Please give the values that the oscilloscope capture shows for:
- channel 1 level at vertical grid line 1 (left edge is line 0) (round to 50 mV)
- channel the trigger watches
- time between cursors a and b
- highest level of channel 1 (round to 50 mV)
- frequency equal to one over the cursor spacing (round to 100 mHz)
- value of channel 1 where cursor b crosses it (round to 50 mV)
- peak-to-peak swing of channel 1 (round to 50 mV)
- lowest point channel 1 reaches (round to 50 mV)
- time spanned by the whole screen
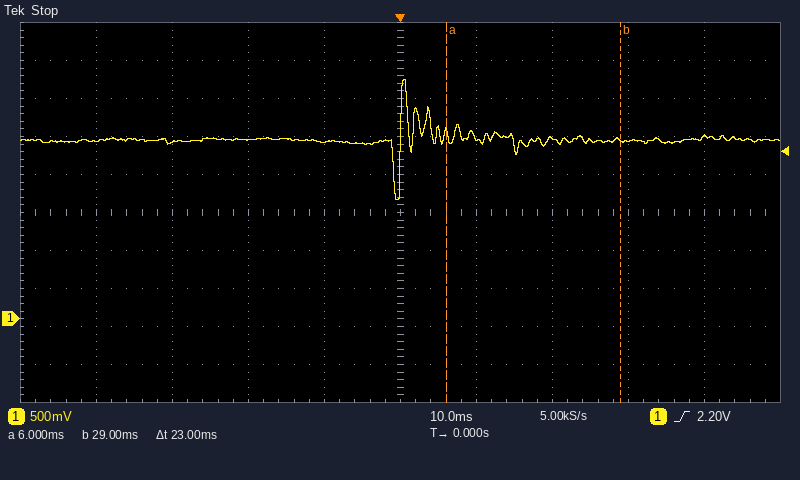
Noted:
2.35 V
channel 1
23 ms
3.15 V
43.5 Hz
2.35 V
1.60 V
1.55 V
100 ms
